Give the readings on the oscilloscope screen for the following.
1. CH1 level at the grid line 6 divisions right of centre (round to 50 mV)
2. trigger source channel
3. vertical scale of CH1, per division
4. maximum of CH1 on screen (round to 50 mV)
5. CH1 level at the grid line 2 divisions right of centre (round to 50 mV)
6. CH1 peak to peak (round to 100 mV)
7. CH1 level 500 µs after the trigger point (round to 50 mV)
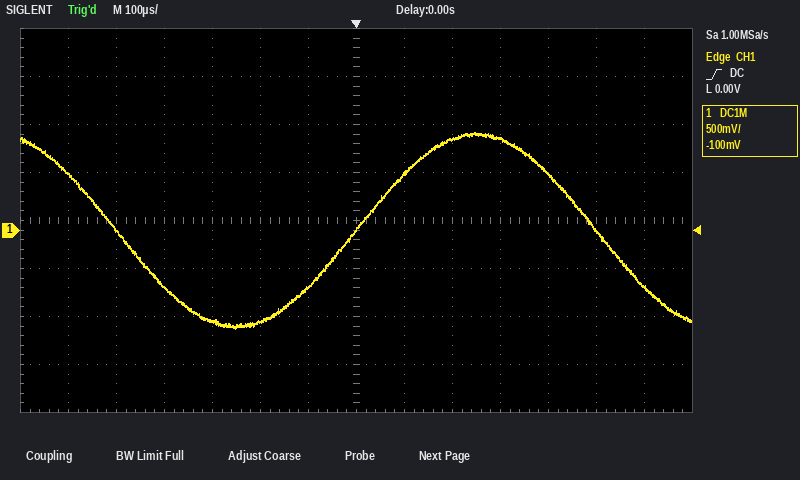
-600 mV
CH1
500 mV
1.00 V
950 mV
2.00 V
0 mV
